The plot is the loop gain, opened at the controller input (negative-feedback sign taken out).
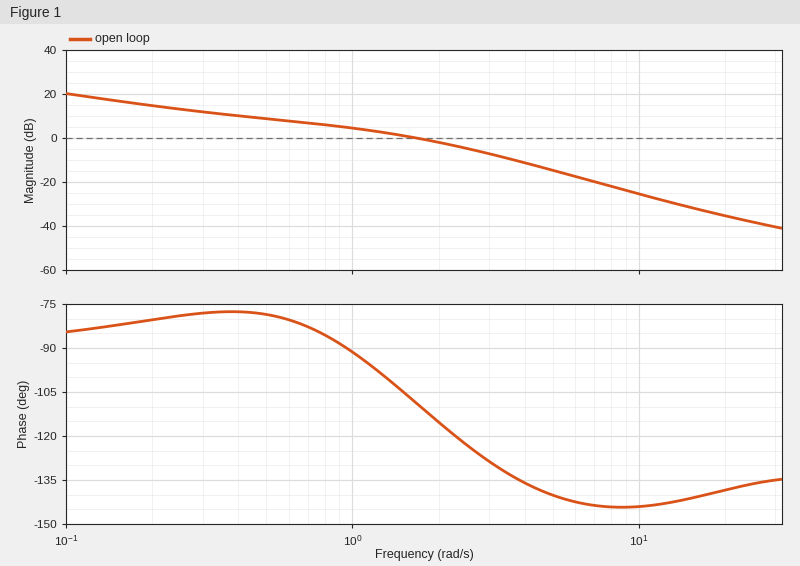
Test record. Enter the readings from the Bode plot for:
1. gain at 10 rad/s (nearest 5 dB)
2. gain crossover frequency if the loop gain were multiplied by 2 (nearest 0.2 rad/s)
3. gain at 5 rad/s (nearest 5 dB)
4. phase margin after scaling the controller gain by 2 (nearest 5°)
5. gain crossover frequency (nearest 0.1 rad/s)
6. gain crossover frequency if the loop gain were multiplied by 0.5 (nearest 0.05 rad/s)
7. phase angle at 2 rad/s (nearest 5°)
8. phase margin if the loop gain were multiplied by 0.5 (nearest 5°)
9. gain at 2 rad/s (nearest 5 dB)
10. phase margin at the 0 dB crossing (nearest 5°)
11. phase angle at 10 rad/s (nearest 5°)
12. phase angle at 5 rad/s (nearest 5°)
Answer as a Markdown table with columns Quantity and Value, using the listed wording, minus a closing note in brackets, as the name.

| Quantity | Value |
|---|---|
| gain at 10 rad/s | -25 dB |
| gain crossover frequency if the loop gain were multiplied by 2 | 2.8 rad/s |
| gain at 5 rad/s | -15 dB |
| phase margin after scaling the controller gain by 2 | 55° |
| gain crossover frequency | 1.7 rad/s |
| gain crossover frequency if the loop gain were multiplied by 0.5 | 0.80 rad/s |
| phase angle at 2 rad/s | -115° |
| phase margin if the loop gain were multiplied by 0.5 | 95° |
| gain at 2 rad/s | 0 dB |
| phase margin at the 0 dB crossing | 70° |
| phase angle at 10 rad/s | -145° |
| phase angle at 5 rad/s | -140° |
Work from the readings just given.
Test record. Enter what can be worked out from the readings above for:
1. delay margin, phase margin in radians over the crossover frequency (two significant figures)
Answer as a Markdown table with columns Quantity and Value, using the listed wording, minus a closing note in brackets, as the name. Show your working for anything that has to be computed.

| Quantity | Value |
|---|---|
| delay margin, phase margin in radians over the crossover frequency | 70 × π / 180 / 1.7 = 0.72 s |
